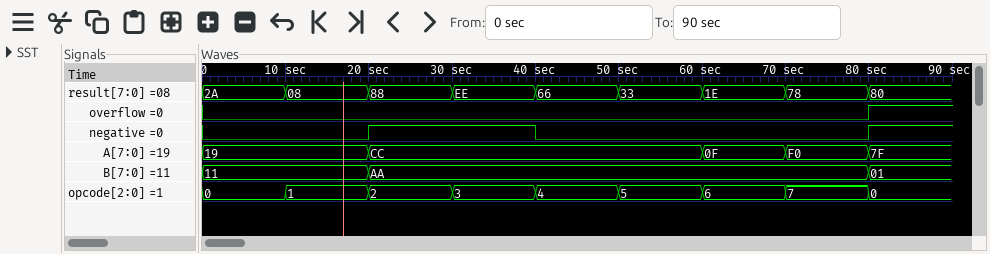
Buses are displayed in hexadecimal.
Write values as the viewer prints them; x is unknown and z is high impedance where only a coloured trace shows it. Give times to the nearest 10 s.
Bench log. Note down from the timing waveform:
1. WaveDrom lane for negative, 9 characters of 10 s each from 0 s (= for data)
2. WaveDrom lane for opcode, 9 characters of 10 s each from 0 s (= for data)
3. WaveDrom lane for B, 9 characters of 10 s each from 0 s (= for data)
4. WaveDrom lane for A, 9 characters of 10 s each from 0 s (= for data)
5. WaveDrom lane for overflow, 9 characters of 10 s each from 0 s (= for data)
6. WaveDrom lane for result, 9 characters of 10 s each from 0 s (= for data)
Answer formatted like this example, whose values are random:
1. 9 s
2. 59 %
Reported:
1. {name: 'negative', wave: '0.1.0...1'}
2. {name: 'opcode', wave: '=========', data: '0 1 2 3 4 5 6 7 0'}
3. {name: 'B', wave: '=.=.....=', data: '11 AA 01'}
4. {name: 'A', wave: '=.=...===', data: '19 CC 0F F0 7F'}
5. {name: 'overflow', wave: '0.......1'}
6. {name: 'result', wave: '=========', data: '2A 08 88 EE 66 33 1E 78 80'}
